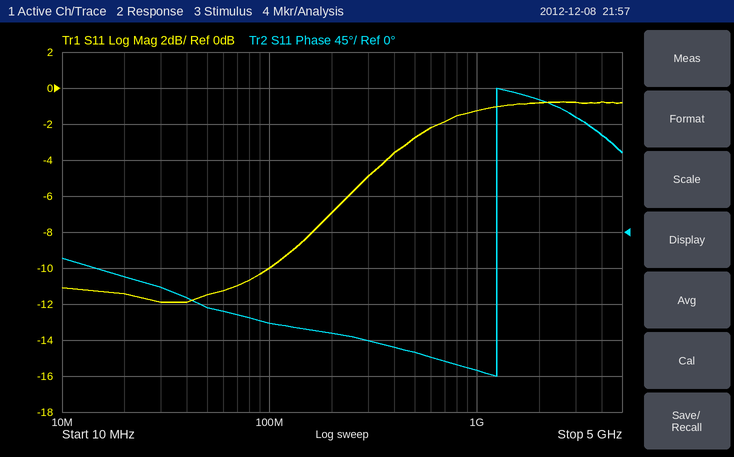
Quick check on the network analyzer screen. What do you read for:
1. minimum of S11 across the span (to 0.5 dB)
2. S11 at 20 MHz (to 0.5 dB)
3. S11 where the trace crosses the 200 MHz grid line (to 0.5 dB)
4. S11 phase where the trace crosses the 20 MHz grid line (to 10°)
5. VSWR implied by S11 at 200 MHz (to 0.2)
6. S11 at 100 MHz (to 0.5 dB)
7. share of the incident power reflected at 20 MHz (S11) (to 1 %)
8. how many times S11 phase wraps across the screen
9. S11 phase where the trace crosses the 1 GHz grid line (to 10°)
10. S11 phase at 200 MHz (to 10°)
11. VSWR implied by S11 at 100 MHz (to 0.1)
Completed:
-12.0 dB
-11.5 dB
-7.0 dB
-60°
2.6
-10.0 dB
7 %
1
-170°
-130°
1.9
